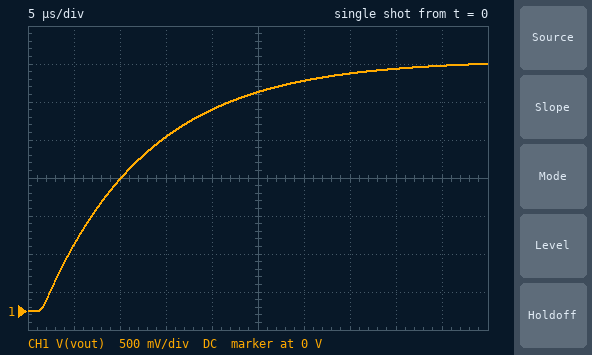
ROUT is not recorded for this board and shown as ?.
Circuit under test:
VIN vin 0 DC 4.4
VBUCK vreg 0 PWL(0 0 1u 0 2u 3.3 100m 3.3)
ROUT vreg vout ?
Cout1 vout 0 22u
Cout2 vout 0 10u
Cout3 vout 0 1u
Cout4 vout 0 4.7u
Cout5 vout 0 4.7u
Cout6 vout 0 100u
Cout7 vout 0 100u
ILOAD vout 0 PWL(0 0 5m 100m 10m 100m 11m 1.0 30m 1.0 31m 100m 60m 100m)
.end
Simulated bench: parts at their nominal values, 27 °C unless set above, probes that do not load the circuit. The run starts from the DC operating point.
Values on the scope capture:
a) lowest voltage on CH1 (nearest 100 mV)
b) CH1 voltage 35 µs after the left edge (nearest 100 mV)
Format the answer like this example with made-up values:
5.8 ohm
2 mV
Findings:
0 V
3.1 V
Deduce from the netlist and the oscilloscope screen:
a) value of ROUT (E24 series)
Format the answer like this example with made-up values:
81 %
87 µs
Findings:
0.047 Ω
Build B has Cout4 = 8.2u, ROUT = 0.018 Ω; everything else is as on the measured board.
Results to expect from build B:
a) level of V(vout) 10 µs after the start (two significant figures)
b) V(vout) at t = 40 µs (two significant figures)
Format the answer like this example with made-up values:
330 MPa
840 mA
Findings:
2.8 V
3.3 V
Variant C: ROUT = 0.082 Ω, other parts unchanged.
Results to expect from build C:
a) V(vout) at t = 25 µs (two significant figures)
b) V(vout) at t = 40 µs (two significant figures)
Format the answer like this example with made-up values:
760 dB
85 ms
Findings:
2.3 V
2.8 V
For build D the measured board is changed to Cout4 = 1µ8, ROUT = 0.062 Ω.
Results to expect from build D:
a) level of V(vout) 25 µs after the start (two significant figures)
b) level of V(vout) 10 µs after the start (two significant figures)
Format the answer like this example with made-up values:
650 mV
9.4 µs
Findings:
2.6 V
1.4 V
